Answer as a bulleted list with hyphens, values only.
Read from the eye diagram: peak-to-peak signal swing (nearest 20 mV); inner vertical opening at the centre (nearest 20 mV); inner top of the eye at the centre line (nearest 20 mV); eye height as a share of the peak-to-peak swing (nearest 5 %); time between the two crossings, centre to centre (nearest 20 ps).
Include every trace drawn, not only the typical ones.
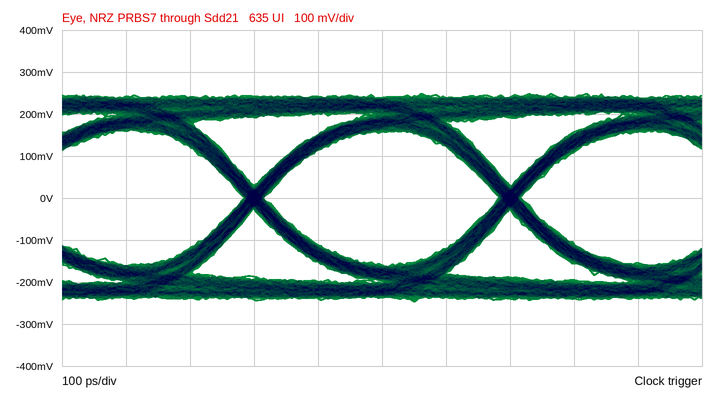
- 500 mV
- 320 mV
- 160 mV
- 65 %
- 400 ps
